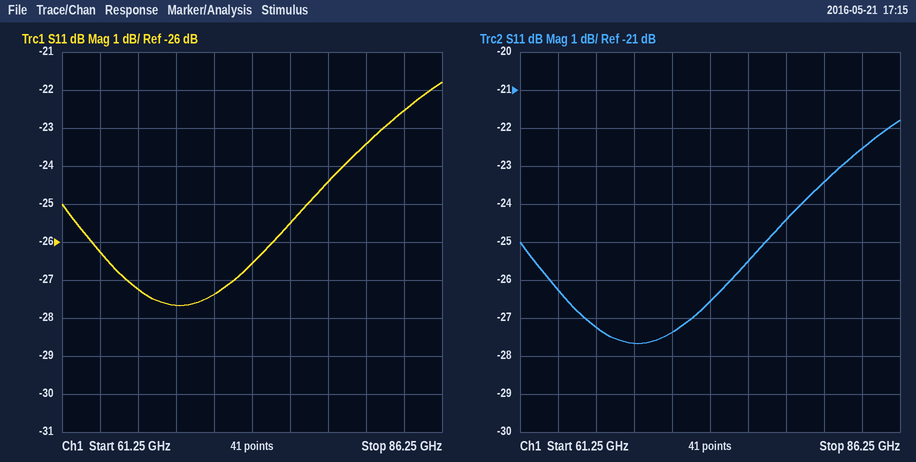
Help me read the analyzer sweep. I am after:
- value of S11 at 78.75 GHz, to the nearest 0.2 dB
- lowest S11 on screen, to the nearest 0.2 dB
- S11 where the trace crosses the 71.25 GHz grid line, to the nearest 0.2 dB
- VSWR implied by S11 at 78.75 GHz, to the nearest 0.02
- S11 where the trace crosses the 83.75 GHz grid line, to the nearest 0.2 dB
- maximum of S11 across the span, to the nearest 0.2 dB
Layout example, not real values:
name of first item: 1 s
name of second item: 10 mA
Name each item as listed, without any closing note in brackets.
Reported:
value of S11 at 78.75 GHz, to the nearest 0.2 dB: -24.4 dB
lowest S11 on screen, to the nearest 0.2 dB: -27.6 dB
S11 where the trace crosses the 71.25 GHz grid line, to the nearest 0.2 dB: -27.4 dB
VSWR implied by S11 at 78.75 GHz, to the nearest 0.02: 1.12
S11 where the trace crosses the 83.75 GHz grid line, to the nearest 0.2 dB: -22.6 dB
maximum of S11 across the span, to the nearest 0.2 dB: -21.8 dB
